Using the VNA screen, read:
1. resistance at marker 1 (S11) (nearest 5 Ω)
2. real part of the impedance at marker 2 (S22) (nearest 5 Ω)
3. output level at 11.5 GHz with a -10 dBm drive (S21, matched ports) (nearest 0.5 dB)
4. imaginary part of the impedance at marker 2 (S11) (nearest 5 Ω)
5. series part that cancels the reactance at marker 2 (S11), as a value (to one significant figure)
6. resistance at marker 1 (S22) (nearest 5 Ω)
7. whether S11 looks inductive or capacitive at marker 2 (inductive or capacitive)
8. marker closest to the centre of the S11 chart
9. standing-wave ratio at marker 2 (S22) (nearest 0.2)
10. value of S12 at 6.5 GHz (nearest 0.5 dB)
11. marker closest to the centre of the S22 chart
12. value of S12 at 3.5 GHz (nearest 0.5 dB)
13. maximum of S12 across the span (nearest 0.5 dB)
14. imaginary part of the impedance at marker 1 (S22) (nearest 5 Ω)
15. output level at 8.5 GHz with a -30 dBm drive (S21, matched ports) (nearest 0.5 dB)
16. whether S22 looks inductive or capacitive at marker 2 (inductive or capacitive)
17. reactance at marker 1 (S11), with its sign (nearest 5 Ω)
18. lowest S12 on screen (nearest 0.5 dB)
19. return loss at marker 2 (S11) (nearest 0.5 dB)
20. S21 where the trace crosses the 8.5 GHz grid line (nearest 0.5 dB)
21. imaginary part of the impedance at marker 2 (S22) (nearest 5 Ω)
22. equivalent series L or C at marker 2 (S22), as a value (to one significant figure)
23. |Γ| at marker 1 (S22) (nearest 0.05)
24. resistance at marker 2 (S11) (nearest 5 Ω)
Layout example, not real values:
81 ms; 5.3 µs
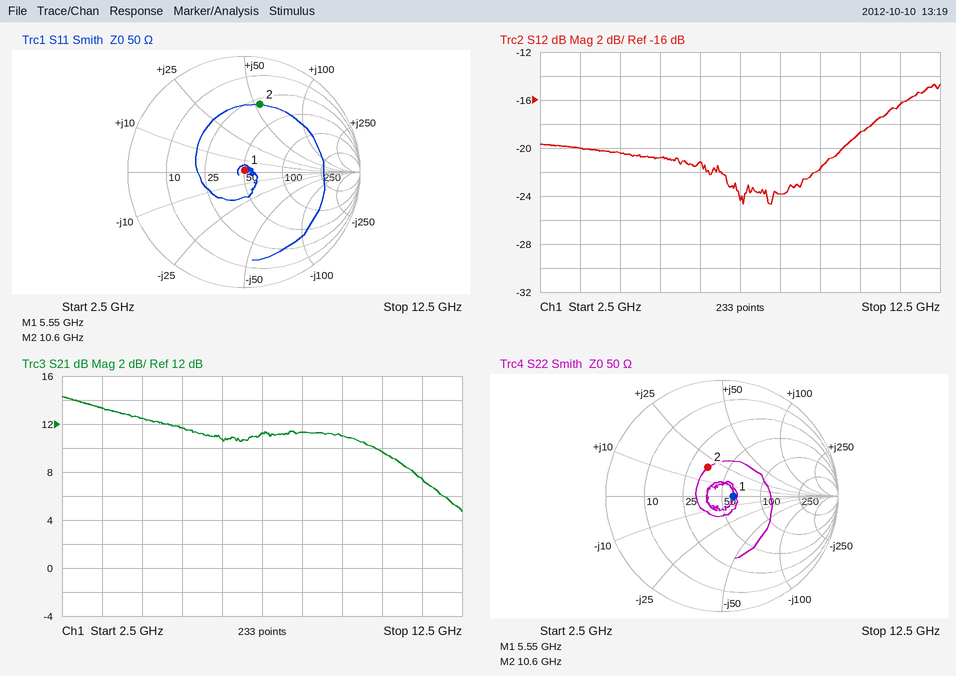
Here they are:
50 Ω; 35 Ω; -2.5 dBm; +55 Ω; 300 fF; 60 Ω; inductive; marker 1; 1.8; -21.0 dB; marker 1; -20.0 dB; -14.5 dB; 0 Ω; -18.5 dBm; inductive; 0 Ω; -24.5 dB; 4.5 dB; 11.5 dB; +20 Ω; 300 pH; 0.10; 30 Ω
